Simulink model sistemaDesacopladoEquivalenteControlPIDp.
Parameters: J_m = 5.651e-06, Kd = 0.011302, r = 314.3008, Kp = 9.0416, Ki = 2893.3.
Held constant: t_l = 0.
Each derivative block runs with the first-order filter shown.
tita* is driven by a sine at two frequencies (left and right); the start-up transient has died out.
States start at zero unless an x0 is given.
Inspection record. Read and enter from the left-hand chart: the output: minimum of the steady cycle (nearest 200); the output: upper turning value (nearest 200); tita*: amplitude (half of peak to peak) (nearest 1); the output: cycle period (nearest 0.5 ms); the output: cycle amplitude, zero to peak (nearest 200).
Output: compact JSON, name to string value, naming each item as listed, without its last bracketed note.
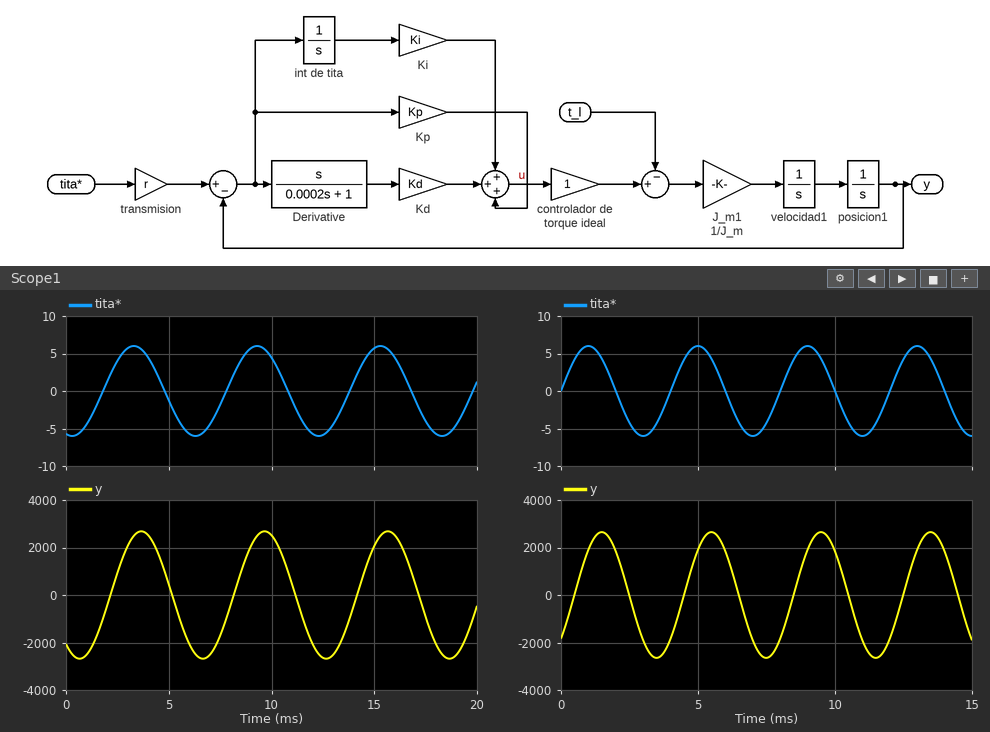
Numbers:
{"the output: minimum of the steady cycle": "-2600", "the output: upper turning value": "2600", "tita*: amplitude (half of peak to peak)": "6", "the output: cycle period": "6.0 ms", "the output: cycle amplitude, zero to peak": "2600"}
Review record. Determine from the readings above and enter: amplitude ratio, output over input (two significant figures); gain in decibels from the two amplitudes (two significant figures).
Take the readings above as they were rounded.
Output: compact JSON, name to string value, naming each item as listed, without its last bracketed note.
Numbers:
{"amplitude ratio, output over input": "430", "gain in decibels from the two amplitudes": "53 dB"}
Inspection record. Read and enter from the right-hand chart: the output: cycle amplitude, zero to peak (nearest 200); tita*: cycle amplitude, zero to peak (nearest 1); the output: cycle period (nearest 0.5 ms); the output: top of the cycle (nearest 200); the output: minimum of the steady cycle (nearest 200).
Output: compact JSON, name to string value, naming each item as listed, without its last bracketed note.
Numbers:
{"the output: cycle amplitude, zero to peak": "2600", "tita*: cycle amplitude, zero to peak": "6", "the output: cycle period": "4.0 ms", "the output: top of the cycle": "2600", "the output: minimum of the steady cycle": "-2600"}
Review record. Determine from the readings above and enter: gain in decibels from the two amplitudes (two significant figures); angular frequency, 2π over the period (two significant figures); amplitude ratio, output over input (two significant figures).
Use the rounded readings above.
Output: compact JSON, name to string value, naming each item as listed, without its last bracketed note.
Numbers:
{"gain in decibels from the two amplitudes": "53 dB", "angular frequency, 2π over the period": "1.6 rad/ms", "amplitude ratio, output over input": "430"}
